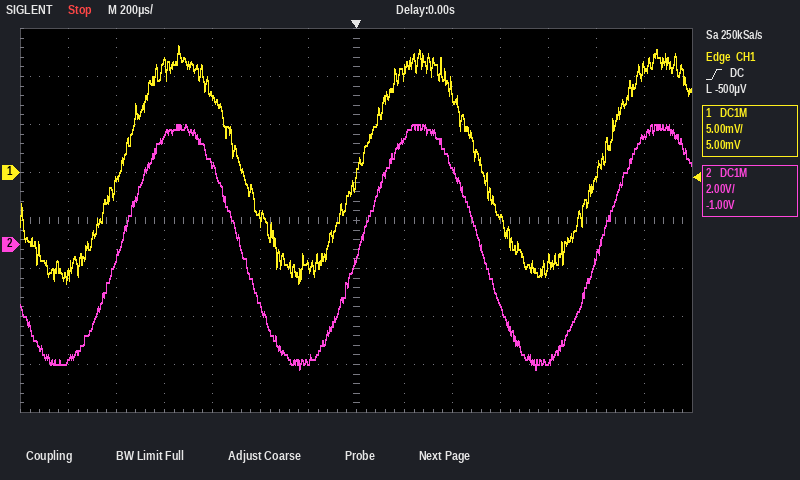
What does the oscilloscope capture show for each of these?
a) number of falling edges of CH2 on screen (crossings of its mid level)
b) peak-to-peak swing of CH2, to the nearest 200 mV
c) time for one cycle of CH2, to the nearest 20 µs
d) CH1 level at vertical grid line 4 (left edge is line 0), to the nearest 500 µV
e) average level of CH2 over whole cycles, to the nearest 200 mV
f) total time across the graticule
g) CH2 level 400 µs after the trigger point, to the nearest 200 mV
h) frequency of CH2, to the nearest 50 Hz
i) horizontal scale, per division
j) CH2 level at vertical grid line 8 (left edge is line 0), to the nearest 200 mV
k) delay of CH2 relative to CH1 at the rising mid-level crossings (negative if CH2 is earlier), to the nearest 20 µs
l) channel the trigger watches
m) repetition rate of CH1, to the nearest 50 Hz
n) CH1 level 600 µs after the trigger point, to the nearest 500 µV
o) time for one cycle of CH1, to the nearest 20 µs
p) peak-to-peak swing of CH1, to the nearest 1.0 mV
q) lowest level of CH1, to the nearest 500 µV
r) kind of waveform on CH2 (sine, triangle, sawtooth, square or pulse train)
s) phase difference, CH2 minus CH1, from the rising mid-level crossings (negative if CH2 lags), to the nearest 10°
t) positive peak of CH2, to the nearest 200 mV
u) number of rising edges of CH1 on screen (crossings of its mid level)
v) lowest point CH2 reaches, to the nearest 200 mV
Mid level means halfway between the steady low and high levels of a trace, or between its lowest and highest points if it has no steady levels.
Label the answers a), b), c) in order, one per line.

a) 2
b) 10.2 V
c) 1.00 ms
d) 8.0 mV
e) 0.0 V
f) 2.8 ms
g) 3.2 V
h) 1.00 kHz
i) 200 µs
j) 4.4 V
k) 0 µs
l) CH1
m) 1.00 kHz
n) -4.5 mV
o) 1.00 ms
p) 25.0 mV
q) -11.5 mV
r) sine
s) 0°
t) 5.0 V
u) 3
v) -5.2 V
